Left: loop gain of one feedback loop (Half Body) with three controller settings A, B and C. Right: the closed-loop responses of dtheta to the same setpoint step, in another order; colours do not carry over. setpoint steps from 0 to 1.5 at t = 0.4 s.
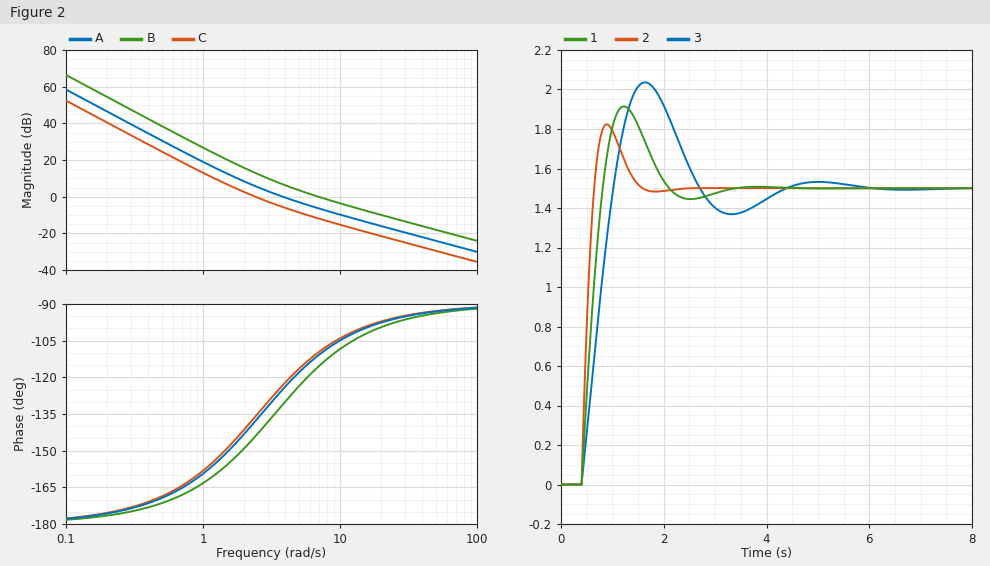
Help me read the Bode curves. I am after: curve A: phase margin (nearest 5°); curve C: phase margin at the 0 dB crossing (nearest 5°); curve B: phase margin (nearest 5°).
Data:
55°
45°
65°
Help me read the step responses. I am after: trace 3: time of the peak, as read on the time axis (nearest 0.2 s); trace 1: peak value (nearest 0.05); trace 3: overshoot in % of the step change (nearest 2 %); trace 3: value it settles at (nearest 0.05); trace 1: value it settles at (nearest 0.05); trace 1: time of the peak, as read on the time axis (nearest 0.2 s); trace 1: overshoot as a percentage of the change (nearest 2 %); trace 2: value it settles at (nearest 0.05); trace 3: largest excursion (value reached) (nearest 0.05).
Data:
1.6 s
1.90
36 %
1.50
1.50
1.2 s
28 %
1.50
2.05
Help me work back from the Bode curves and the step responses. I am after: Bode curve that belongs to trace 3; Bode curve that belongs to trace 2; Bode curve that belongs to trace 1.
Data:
C
B
A
